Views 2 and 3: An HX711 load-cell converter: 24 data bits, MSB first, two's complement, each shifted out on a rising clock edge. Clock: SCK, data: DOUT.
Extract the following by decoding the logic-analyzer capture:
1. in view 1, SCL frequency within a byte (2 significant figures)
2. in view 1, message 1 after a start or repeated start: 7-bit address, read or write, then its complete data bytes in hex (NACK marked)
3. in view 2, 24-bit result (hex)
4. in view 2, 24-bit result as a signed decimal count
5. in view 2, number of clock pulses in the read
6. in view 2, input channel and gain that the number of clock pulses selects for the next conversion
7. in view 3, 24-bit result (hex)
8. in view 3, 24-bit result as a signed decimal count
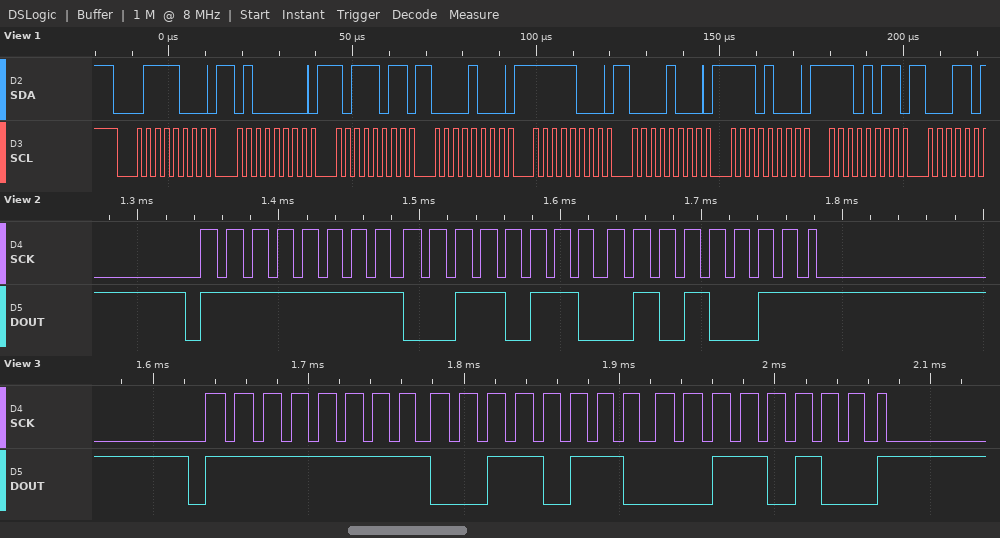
400 kHz
0x3C write: 40 BB 08 F8 08 E8 EB
0xFF3653
-51629
25
channel A, gain 128
0xFF3634
-51660
